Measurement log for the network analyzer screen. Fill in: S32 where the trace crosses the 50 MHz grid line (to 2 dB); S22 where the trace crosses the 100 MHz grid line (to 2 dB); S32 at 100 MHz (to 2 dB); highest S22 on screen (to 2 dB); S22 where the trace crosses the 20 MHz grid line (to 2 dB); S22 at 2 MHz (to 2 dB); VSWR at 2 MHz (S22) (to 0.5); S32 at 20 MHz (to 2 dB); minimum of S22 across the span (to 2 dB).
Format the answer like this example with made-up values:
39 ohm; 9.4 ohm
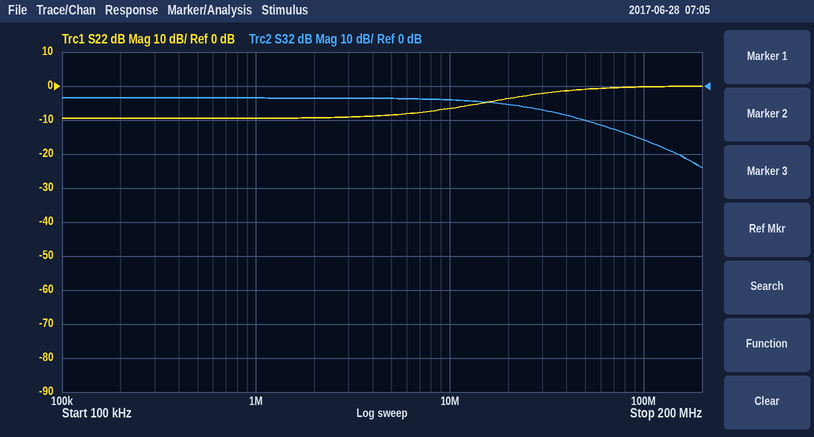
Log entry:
-10 dB; 0 dB; -16 dB; 0 dB; -4 dB; -10 dB; 2.0; -6 dB; -10 dB
